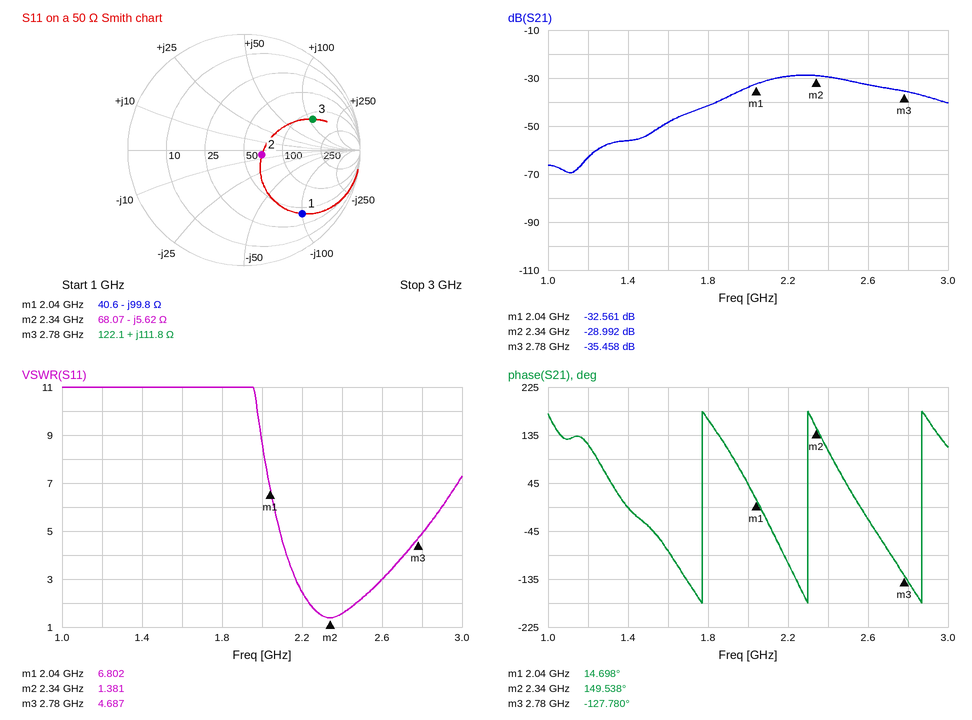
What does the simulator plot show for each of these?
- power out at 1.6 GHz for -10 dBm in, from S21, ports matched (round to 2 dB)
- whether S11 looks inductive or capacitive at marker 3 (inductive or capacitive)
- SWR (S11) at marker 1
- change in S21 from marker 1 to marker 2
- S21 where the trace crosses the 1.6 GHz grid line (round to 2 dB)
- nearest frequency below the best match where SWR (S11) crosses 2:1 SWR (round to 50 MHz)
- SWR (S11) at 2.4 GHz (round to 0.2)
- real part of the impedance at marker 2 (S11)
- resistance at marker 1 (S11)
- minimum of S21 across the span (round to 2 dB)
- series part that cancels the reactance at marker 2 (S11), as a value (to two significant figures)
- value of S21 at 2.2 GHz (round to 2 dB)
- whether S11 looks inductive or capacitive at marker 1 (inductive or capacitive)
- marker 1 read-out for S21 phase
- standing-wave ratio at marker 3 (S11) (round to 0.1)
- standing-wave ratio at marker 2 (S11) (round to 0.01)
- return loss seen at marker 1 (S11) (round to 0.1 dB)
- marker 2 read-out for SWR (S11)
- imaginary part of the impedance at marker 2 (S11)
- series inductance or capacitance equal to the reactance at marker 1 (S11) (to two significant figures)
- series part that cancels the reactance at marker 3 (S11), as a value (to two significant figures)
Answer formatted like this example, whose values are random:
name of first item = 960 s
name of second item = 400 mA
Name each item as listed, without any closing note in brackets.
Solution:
power out at 1.6 GHz for -10 dBm in, from S21, ports matched = -58 dBm
whether S11 looks inductive or capacitive at marker 3 = inductive
SWR (S11) at marker 1 = 6.802
change in S21 from marker 1 to marker 2 = 3.569 dB
S21 where the trace crosses the 1.6 GHz grid line = -48 dB
nearest frequency below the best match where SWR (S11) crosses 2:1 SWR = 2.25 GHz
SWR (S11) at 2.4 GHz = 1.6
real part of the impedance at marker 2 = 68.07 Ω
resistance at marker 1 = 40.6 Ω
minimum of S21 across the span = -70 dB
series part that cancels the reactance at marker 2 (S11), as a value = 380 pH
value of S21 at 2.2 GHz = -30 dB
whether S11 looks inductive or capacitive at marker 1 = capacitive
marker 1 read-out for S21 phase = 14.698°
standing-wave ratio at marker 3 (S11) = 4.7
standing-wave ratio at marker 2 (S11) = 1.38
return loss seen at marker 1 (S11) = 2.6 dB
marker 2 read-out for SWR = 1.381
imaginary part of the impedance at marker 2 = -5.62 Ω
series inductance or capacitance equal to the reactance at marker 1 (S11) = 780 fF
series part that cancels the reactance at marker 3 (S11), as a value = 510 fF
